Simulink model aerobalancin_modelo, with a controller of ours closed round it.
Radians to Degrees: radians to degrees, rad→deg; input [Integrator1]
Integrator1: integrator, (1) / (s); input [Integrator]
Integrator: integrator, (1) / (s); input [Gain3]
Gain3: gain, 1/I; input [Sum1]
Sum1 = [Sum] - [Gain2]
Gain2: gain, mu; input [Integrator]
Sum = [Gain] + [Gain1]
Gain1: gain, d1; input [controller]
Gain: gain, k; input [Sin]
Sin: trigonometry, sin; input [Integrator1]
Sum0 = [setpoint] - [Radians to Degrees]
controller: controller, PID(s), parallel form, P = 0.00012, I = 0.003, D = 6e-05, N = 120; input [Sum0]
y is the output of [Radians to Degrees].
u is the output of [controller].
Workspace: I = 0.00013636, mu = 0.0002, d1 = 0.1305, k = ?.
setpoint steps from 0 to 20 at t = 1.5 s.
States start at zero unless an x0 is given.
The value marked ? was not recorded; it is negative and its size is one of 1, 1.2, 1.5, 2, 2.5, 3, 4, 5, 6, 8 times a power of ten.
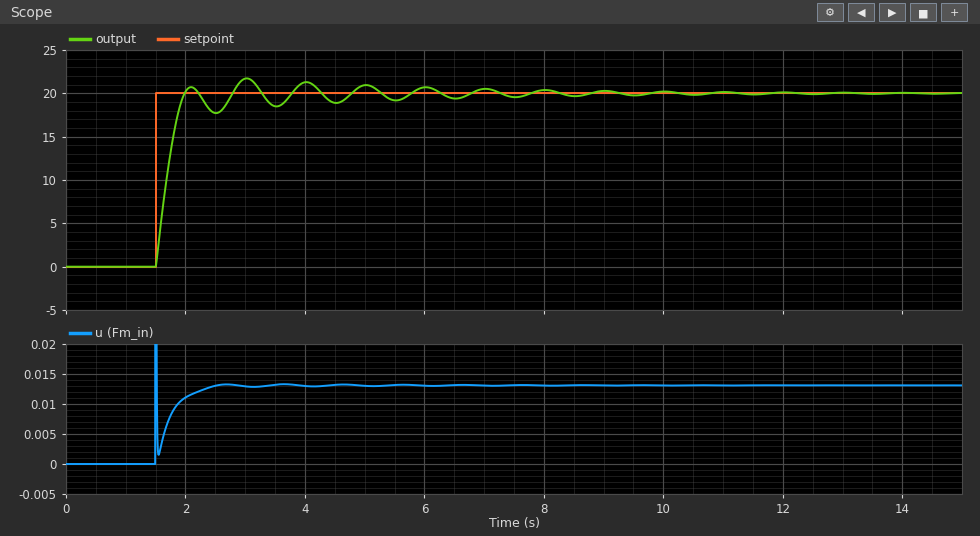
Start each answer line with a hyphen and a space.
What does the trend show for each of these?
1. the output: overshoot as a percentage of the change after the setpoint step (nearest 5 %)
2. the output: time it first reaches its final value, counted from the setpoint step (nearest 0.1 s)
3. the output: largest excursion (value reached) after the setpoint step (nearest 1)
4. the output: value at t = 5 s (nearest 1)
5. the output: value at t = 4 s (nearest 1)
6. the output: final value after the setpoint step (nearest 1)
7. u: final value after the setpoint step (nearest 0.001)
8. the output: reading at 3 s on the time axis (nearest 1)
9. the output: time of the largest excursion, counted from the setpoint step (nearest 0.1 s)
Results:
- 10 %
- 0.5 s
- 22
- 21
- 21
- 20
- 0.013
- 22
- 1.5 s
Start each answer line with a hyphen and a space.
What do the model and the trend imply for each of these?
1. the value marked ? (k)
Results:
- -0.005
